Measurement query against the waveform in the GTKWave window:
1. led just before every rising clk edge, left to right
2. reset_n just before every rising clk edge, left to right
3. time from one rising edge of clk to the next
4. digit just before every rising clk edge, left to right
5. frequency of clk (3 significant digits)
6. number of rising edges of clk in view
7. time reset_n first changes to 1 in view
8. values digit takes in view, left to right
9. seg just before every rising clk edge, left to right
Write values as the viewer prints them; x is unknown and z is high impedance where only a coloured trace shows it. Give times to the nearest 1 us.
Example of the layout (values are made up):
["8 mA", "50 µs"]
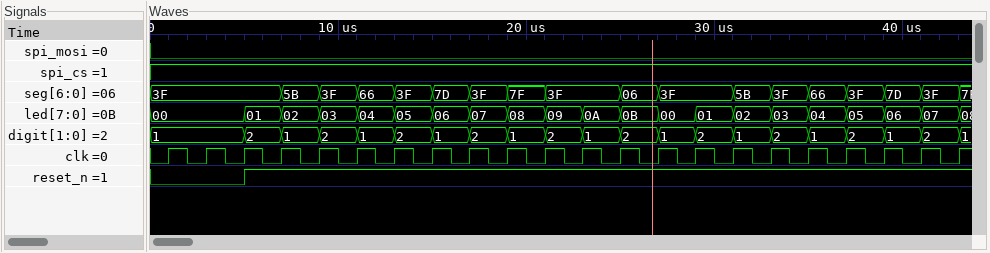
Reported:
["00, 00, 00, 01, 02, 03, 04, 05, 06, 07, 08, 09, 0A, 0B, 00, 01, 02, 03, 04, 05, 06, 07", "0 0 0 1 1 1 1 1 1 1 1 1 1 1 1 1 1 1 1 1 1 1", "2 us", "1, 1, 1, 2, 1, 2, 1, 2, 1, 2, 1, 2, 1, 2, 1, 2, 1, 2, 1, 2, 1, 2", "500 kHz", "22", "5 us", "1, 2, 1, 2, 1, 2, 1, 2, 1, 2, 1, 2, 1, 2, 1, 2, 1, 2, 1, 2, 1", "3F, 3F, 3F, 3F, 5B, 3F, 66, 3F, 7D, 3F, 7F, 3F, 3F, 06, 3F, 3F, 5B, 3F, 66, 3F, 7D, 3F"]
